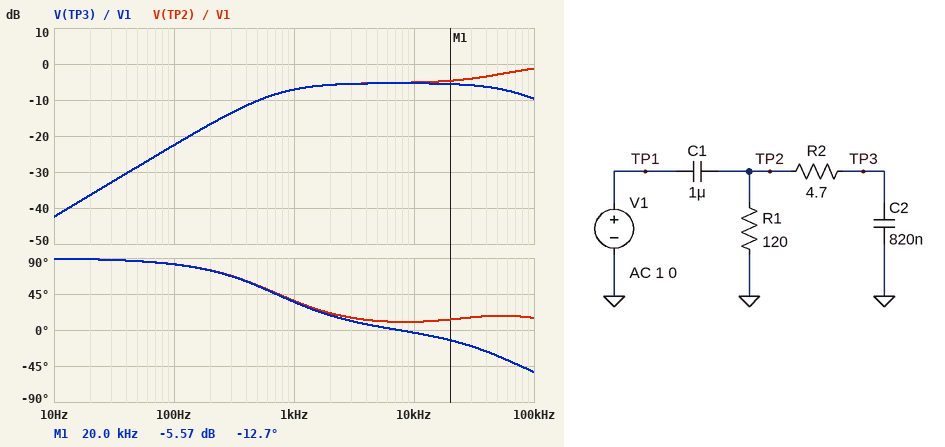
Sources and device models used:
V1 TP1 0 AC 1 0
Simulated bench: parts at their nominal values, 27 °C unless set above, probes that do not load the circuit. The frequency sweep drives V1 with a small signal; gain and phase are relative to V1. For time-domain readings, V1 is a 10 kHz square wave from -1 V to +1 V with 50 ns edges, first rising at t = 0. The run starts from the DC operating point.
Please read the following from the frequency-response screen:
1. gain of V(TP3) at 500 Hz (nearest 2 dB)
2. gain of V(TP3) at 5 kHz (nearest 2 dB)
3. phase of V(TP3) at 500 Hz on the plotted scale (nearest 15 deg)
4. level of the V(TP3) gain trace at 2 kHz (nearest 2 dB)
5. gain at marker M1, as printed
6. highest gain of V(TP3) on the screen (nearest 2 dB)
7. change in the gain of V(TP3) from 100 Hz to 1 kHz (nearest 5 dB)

-10 dB
-6 dB
60 deg
-6 dB
-5.57 dB
-6 dB
15 dB
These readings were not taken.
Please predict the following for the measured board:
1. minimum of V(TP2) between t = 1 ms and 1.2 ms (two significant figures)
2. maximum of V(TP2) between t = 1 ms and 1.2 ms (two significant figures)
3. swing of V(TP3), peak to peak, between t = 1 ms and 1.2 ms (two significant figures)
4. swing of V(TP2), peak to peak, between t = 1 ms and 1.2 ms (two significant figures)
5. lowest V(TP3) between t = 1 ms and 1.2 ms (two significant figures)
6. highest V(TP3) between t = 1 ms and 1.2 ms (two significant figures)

-1.5 V
1.5 V
1.2 V
3.0 V
-570 mV
580 mV
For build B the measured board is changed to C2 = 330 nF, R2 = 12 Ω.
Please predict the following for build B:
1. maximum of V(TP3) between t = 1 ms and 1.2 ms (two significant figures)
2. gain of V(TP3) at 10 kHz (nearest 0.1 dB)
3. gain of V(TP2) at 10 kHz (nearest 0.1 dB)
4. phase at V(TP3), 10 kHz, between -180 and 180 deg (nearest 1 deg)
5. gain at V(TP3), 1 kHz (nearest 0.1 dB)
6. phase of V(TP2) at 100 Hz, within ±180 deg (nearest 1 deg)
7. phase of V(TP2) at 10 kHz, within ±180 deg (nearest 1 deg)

790 mV
-2.7 dB
-2.5 dB
-5 deg
-5.5 dB
84 deg
9 deg
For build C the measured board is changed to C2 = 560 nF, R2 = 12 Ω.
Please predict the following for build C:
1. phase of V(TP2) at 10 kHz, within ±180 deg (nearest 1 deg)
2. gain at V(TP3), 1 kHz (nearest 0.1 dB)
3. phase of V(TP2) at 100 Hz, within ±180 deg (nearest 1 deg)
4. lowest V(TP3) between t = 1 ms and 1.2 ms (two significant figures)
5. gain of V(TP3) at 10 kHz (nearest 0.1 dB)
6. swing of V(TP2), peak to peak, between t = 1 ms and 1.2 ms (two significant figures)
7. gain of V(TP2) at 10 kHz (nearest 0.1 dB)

13 deg
-6.3 dB
83 deg
-650 mV
-4.3 dB
2.9 V
-3.6 dB
